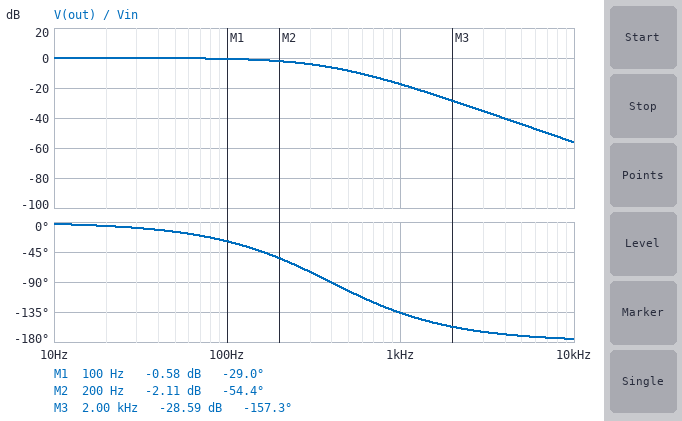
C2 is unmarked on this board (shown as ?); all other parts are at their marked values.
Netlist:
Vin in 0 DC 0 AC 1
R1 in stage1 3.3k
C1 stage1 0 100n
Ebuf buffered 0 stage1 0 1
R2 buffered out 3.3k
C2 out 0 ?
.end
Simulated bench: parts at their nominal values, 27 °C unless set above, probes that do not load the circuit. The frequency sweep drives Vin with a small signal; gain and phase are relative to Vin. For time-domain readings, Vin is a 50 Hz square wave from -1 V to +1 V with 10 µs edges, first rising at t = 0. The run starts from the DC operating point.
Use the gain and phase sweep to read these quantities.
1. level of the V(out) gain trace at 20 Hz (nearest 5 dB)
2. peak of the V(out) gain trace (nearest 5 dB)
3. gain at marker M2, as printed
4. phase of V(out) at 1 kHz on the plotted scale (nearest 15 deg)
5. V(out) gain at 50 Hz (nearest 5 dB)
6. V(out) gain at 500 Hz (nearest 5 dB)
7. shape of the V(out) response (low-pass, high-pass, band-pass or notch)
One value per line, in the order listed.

0 dB
0 dB
-2.11 dB
-135 deg
0 dB
-10 dB
low-pass
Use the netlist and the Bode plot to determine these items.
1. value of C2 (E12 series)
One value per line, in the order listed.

150 nF
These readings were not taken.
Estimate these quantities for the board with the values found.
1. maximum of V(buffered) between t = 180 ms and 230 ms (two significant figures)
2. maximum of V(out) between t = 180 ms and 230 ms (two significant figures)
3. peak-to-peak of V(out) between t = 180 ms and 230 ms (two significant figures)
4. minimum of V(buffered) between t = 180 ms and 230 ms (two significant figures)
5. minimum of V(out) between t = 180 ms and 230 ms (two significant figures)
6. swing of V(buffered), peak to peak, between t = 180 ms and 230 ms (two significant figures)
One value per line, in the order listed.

1.0 V
1.0 V
2.0 V
-1.0 V
-1.0 V
2.0 V
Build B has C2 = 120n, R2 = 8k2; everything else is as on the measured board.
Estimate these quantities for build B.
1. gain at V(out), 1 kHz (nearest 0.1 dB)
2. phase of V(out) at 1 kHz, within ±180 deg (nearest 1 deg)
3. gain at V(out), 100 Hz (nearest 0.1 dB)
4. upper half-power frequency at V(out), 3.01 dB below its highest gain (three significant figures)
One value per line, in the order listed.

-23.2 dB
-145 deg
-1.6 dB
147 Hz
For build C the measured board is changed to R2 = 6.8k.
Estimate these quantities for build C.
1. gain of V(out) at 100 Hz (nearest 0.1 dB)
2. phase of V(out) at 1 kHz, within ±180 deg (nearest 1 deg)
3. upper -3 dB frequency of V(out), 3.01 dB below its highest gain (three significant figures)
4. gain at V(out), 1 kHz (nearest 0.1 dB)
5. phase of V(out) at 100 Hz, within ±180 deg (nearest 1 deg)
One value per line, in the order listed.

-1.7 dB
-145 deg
143 Hz
-23.5 dB
-44 deg
